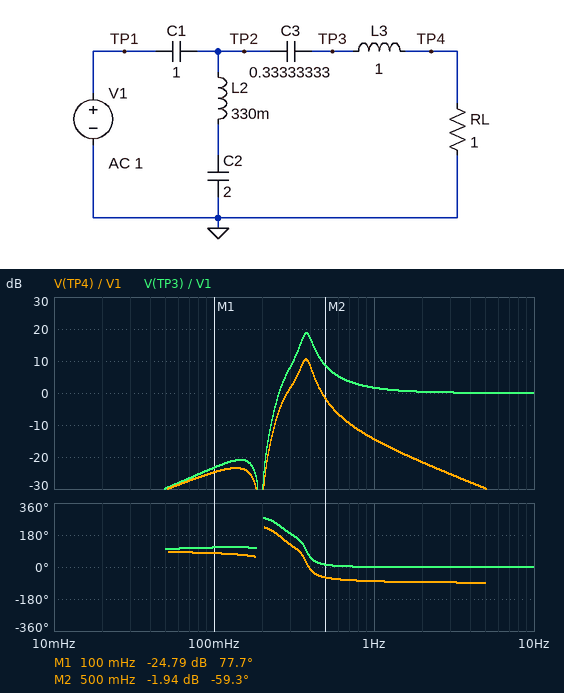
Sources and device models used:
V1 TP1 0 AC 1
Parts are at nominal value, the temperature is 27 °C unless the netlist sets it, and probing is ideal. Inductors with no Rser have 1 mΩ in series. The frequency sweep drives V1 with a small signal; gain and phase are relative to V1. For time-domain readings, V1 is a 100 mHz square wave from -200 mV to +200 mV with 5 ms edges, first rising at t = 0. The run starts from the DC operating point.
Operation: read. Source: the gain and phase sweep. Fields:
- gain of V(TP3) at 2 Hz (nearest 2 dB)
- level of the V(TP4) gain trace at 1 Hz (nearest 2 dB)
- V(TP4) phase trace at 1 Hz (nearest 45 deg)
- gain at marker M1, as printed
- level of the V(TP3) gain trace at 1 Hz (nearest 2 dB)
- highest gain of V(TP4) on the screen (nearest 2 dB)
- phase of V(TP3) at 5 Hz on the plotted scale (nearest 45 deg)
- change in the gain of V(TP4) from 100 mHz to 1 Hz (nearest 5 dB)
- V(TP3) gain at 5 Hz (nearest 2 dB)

0 dB
-14 dB
-90 deg
-24.79 dB
2 dB
10 dB
0 deg
10 dB
0 dB
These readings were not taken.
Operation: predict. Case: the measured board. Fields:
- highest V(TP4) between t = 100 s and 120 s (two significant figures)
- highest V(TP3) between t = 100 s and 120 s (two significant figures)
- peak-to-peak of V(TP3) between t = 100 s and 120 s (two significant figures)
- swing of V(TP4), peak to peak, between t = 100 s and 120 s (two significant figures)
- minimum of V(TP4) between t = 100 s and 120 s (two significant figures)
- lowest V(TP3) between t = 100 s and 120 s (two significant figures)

130 mV
310 mV
630 mV
260 mV
-130 mV
-310 mV
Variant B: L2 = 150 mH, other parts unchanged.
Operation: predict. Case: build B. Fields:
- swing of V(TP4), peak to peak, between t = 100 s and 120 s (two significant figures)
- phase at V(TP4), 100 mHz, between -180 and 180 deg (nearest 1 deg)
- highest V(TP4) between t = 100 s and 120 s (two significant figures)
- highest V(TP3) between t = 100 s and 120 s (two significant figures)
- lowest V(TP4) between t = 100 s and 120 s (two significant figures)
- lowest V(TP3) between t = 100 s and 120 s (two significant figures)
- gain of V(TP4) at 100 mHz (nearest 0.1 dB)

330 mV
78 deg
160 mV
530 mV
-160 mV
-530 mV
-23.8 dB
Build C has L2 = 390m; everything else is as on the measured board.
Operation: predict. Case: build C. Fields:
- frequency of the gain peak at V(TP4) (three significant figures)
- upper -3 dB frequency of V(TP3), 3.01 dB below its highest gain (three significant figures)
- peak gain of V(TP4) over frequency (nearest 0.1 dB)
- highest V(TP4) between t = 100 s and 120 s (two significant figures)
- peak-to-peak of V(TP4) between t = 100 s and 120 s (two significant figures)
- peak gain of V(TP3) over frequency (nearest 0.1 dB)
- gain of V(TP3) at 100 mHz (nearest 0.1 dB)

355 mHz
400 mHz
9.0 dB
160 mV
330 mV
16.8 dB
-23.7 dB
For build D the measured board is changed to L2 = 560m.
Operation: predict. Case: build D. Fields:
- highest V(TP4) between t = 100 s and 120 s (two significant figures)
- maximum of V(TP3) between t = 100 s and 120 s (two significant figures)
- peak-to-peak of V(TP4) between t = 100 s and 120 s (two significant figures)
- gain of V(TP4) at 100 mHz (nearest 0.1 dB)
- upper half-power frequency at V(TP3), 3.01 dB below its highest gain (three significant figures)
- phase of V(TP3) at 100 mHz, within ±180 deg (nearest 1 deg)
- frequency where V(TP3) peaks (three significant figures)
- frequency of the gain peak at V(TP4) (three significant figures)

190 mV
540 mV
390 mV
-26.5 dB
403 mHz
110 deg
336 mHz
326 mHz
